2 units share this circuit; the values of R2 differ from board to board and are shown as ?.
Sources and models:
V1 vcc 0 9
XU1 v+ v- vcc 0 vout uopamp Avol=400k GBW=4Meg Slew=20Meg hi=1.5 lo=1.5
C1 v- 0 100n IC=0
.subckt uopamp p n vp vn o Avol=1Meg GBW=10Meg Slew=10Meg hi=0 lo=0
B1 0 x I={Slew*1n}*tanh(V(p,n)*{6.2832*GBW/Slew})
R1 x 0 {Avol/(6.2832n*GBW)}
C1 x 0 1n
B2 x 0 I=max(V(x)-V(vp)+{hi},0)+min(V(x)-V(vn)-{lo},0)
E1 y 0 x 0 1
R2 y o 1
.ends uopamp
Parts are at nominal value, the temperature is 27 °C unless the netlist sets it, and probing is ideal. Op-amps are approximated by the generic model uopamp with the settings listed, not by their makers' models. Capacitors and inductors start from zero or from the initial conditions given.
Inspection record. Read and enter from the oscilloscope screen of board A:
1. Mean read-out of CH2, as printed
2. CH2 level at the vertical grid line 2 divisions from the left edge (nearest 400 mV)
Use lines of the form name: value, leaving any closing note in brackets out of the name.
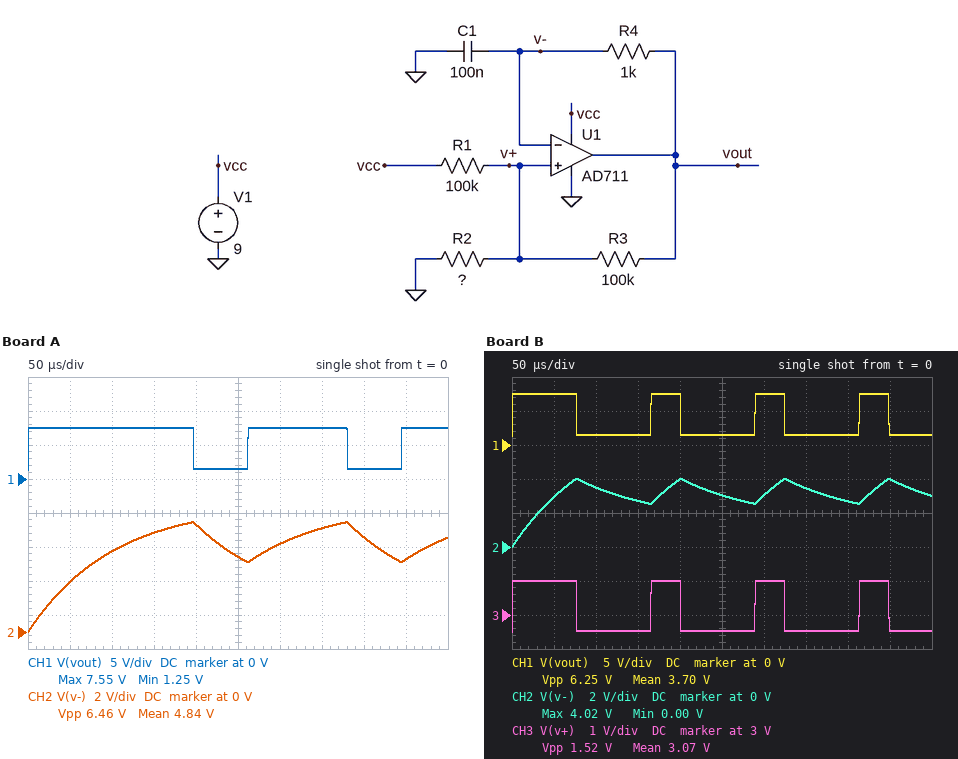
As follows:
Mean read-out of CH2, as printed: 4.84 V
CH2 level at the vertical grid line 2 divisions from the left edge: 4.8 V
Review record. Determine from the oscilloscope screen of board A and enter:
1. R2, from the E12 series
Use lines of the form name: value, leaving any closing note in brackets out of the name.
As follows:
R2, from the E12 series: 180 kΩ
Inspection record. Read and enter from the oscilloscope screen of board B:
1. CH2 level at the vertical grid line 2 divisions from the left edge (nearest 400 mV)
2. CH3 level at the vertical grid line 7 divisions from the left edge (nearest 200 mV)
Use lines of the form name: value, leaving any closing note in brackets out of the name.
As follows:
CH2 level at the vertical grid line 2 divisions from the left edge: 3.6 V
CH3 level at the vertical grid line 7 divisions from the left edge: 2.6 V
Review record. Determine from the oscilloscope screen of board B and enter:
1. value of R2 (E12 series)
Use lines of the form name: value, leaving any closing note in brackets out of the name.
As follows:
value of R2: 47 kΩ
